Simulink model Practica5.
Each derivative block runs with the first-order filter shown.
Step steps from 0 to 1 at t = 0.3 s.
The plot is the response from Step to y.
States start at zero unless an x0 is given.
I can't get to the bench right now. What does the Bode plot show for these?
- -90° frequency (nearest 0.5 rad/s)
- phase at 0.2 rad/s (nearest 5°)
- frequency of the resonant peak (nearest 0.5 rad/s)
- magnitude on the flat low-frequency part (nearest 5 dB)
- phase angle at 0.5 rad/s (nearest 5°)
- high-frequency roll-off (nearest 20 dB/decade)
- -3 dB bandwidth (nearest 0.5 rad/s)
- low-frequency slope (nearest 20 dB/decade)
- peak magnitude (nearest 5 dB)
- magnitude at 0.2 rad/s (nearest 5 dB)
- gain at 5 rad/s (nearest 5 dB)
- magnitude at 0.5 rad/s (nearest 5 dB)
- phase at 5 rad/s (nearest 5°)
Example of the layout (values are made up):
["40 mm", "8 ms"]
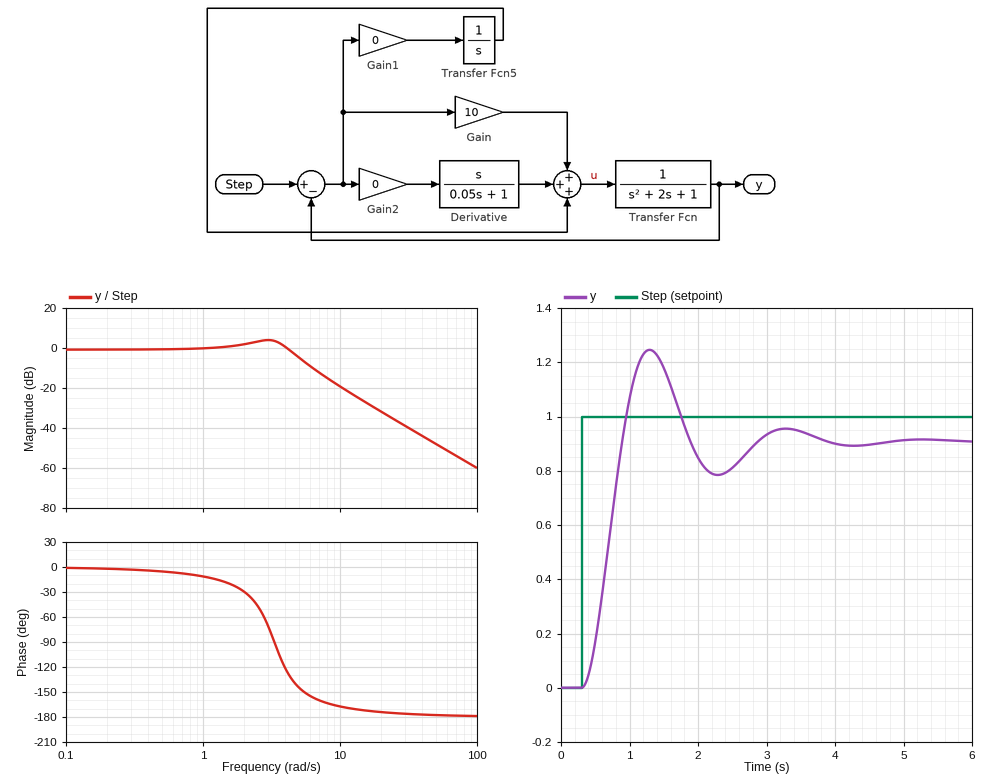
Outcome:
["3.5 rad/s", "0°", "3.0 rad/s", "0 dB", "-5°", "-40 dB/decade", "5.0 rad/s", "0 dB/decade", "5 dB", "0 dB", "-5 dB", "0 dB", "-145°"]
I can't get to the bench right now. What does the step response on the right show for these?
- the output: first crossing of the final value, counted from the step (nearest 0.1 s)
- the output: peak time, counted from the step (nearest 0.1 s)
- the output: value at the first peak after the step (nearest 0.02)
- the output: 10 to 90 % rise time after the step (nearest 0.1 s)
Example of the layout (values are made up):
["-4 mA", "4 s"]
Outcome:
["0.6 s", "1.0 s", "1.24", "0.4 s"]
